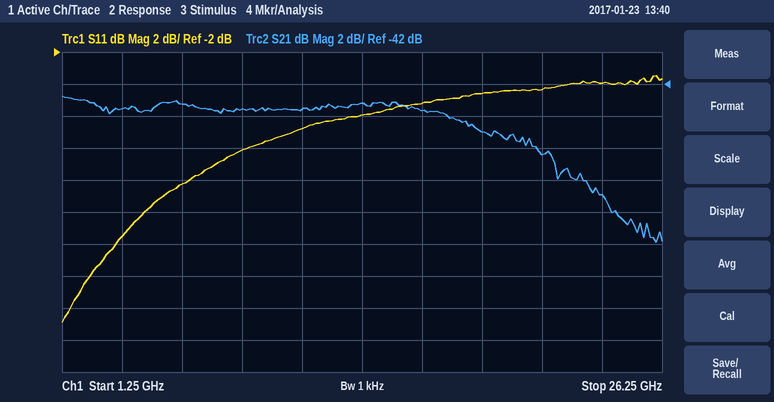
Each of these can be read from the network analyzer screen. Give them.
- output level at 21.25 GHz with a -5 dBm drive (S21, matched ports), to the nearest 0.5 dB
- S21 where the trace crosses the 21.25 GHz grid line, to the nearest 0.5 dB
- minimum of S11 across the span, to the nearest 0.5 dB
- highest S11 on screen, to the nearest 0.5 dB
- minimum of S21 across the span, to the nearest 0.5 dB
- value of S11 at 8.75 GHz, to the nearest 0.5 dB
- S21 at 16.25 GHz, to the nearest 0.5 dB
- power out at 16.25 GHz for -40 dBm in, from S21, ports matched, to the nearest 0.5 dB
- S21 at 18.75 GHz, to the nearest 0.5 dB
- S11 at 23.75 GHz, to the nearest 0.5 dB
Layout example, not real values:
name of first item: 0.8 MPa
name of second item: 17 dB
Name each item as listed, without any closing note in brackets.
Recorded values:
output level at 21.25 GHz with a -5 dBm drive (S21, matched ports), to the nearest 0.5 dB: -51.5 dBm
S21 where the trace crosses the 21.25 GHz grid line, to the nearest 0.5 dB: -46.5 dB
minimum of S11 across the span, to the nearest 0.5 dB: -19.0 dB
highest S11 on screen, to the nearest 0.5 dB: -3.5 dB
minimum of S21 across the span, to the nearest 0.5 dB: -52.0 dB
value of S11 at 8.75 GHz, to the nearest 0.5 dB: -8.0 dB
S21 at 16.25 GHz, to the nearest 0.5 dB: -43.5 dB
power out at 16.25 GHz for -40 dBm in, from S21, ports matched, to the nearest 0.5 dB: -83.5 dBm
S21 at 18.75 GHz, to the nearest 0.5 dB: -45.0 dB
S11 at 23.75 GHz, to the nearest 0.5 dB: -4.0 dB
